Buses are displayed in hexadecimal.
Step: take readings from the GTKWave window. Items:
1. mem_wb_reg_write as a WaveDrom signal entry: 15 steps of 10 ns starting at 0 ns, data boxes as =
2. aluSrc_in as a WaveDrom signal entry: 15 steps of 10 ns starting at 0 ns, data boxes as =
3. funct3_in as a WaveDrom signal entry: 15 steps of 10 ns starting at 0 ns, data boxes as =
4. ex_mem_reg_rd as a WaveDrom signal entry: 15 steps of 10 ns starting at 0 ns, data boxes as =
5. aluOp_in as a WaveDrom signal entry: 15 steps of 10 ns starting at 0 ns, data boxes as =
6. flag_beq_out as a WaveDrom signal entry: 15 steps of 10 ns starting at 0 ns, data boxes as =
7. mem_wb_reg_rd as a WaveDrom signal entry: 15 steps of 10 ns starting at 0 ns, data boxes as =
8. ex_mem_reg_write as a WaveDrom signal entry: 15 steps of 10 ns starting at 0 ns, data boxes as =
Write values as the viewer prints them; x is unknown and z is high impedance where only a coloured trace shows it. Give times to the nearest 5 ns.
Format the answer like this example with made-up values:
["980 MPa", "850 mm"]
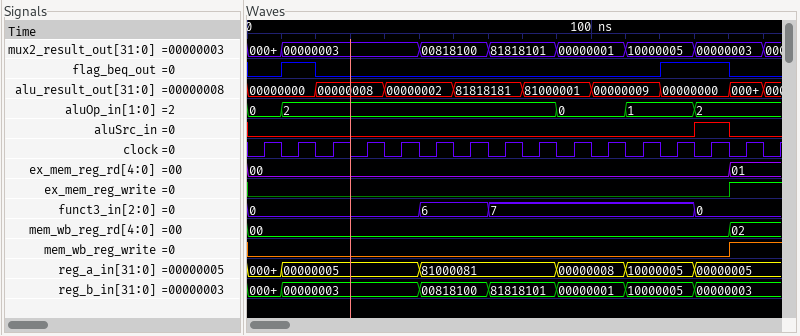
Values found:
["{name: 'mem_wb_reg_write', wave: '0.............1'}", "{name: 'aluSrc_in', wave: '0............10'}", "{name: 'funct3_in', wave: '=....=.=.....=.', data: '0 6 7 0'}", "{name: 'ex_mem_reg_rd', wave: '=.............=', data: '00 01'}", "{name: 'aluOp_in', wave: '==.......=.=.=.', data: '0 2 0 1 2'}", "{name: 'flag_beq_out', wave: '010.........1.0'}", "{name: 'mem_wb_reg_rd', wave: '=.............=', data: '00 02'}", "{name: 'ex_mem_reg_write', wave: '0.............1'}"]
